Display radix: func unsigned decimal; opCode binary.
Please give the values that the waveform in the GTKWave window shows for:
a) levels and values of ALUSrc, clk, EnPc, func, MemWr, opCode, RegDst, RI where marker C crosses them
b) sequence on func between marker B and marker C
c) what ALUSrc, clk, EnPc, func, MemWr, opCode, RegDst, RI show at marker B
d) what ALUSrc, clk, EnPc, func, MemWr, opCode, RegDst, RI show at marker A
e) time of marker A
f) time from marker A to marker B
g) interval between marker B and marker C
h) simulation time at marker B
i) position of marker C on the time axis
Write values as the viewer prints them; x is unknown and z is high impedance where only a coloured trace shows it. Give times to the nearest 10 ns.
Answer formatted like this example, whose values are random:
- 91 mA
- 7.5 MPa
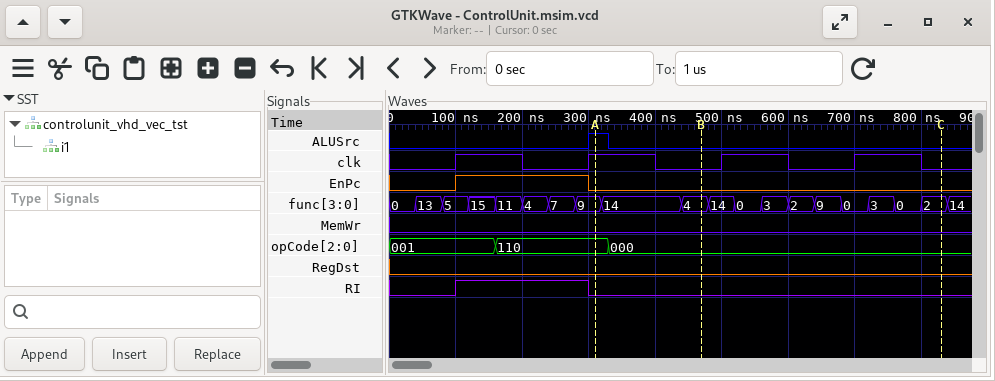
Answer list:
- ALUSrc=0, clk=0, EnPc=0, func=2, MemWr=0, opCode=000, RegDst=0, RI=0
- 4, 14, 0, 3, 2, 9, 0, 3, 0, 2
- ALUSrc=0, clk=0, EnPc=0, func=4, MemWr=0, opCode=000, RegDst=0, RI=0
- ALUSrc=1, clk=1, EnPc=0, func=9, MemWr=0, opCode=110, RegDst=0, RI=0
- 310 ns
- 160 ns
- 360 ns
- 470 ns
- 830 ns
